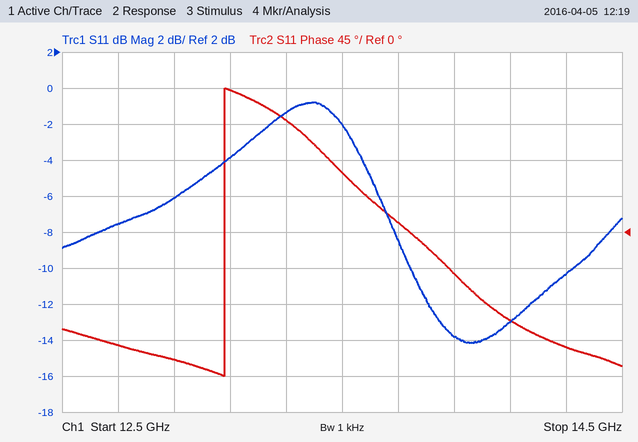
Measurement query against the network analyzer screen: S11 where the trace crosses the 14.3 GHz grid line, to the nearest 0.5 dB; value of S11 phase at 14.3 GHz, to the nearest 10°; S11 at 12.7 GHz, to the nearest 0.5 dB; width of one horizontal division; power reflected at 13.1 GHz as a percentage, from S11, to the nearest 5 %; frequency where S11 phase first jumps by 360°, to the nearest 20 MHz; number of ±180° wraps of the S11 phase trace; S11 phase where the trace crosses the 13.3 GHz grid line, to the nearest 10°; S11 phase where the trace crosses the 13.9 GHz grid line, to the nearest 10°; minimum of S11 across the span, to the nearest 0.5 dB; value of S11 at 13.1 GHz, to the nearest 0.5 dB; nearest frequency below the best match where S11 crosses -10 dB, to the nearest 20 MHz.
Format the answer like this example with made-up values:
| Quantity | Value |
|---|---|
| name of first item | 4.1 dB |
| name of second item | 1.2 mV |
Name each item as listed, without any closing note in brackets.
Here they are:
| Quantity | Value |
|---|---|
| S11 where the trace crosses the 14.3 GHz grid line, to the nearest 0.5 dB | -10.5 dB |
| value of S11 phase at 14.3 GHz, to the nearest 10° | -140° |
| S11 at 12.7 GHz, to the nearest 0.5 dB | -7.5 dB |
| width of one horizontal division | 200 MHz |
| power reflected at 13.1 GHz as a percentage, from S11, to the nearest 5 % | 40 % |
| frequency where S11 phase first jumps by 360°, to the nearest 20 MHz | 13.08 GHz |
| number of ±180° wraps of the S11 phase trace | 1 |
| S11 phase where the trace crosses the 13.3 GHz grid line, to the nearest 10° | 140° |
| S11 phase where the trace crosses the 13.9 GHz grid line, to the nearest 10° | -50° |
| minimum of S11 across the span, to the nearest 0.5 dB | -14.0 dB |
| value of S11 at 13.1 GHz, to the nearest 0.5 dB | -4.0 dB |
| nearest frequency below the best match where S11 crosses -10 dB, to the nearest 20 MHz | 13.74 GHz |
